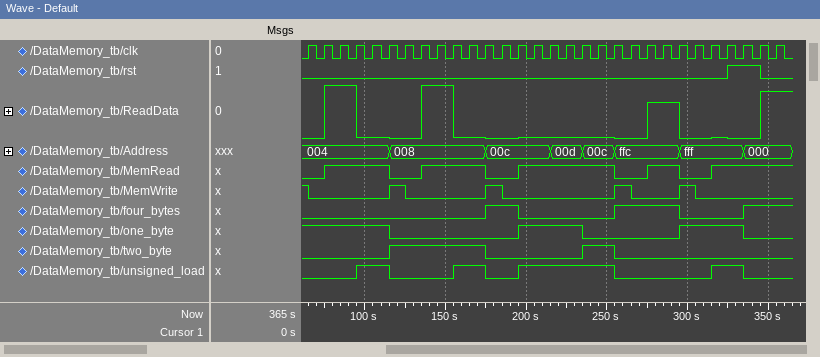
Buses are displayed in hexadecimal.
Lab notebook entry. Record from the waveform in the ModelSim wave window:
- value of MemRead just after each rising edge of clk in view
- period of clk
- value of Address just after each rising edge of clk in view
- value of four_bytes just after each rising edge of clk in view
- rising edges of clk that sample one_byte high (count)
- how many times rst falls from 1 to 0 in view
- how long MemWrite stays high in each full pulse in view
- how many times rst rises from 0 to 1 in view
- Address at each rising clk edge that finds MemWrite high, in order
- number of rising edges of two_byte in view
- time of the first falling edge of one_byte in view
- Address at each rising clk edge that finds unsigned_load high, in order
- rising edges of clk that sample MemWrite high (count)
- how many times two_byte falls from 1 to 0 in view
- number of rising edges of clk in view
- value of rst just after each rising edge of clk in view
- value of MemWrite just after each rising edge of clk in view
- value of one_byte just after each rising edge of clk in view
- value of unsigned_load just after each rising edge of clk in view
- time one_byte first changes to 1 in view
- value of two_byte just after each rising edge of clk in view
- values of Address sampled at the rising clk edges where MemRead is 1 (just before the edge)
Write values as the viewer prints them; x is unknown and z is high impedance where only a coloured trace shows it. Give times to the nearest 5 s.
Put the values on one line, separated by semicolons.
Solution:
0 1 1 1 1 0 0 1 1 1 1 0 0 1 1 1 1 1 1 0 0 1 1 0 0 1 1 1 1 1; 10 s; 004, 004, 004, 004, 004, 008, 008, 008, 008, 008, 008, 00c, 00c, 00c, 00c, 00d, 00d, 00c, 00c, ffc, ffc, ffc, ffc, fff, fff, fff, fff, 000, 000, 000; 0 0 0 0 0 0 0 0 0 0 0 1 1 0 0 0 0 0 0 1 1 1 1 0 0 0 0 1 1 1; 14; 1; 10 s, 10 s, 10 s, 10 s; 1; 004, 008, 00c, ffc, fff; 2; 115 s; 004, 004, 008, 008, 00c, 00c, 00d, 00d, 00c, 00c, fff, fff; 5; 2; 30; 0 0 0 0 0 0 0 0 0 0 0 0 0 0 0 0 0 0 0 0 0 0 0 0 0 0 1 1 0 0; 0 0 0 0 0 1 0 0 0 0 0 1 0 0 0 0 0 0 0 1 0 0 0 1 0 0 0 0 0 0; 1 1 1 1 1 0 0 0 0 0 0 0 0 1 1 1 1 0 0 0 0 0 0 1 1 1 1 0 0 0; 0 0 0 1 1 0 0 0 0 1 1 0 0 1 1 1 1 1 1 0 0 0 0 0 0 1 1 0 0 0; 195 s; 0 0 0 0 0 1 1 1 1 1 1 0 0 0 0 0 0 1 1 0 0 0 0 0 0 0 0 0 0 0; 004, 004, 004, 004, 008, 008, 008, 008, 00c, 00c, 00d, 00d, 00c, 00c, ffc, ffc, fff, fff, 000, 000
